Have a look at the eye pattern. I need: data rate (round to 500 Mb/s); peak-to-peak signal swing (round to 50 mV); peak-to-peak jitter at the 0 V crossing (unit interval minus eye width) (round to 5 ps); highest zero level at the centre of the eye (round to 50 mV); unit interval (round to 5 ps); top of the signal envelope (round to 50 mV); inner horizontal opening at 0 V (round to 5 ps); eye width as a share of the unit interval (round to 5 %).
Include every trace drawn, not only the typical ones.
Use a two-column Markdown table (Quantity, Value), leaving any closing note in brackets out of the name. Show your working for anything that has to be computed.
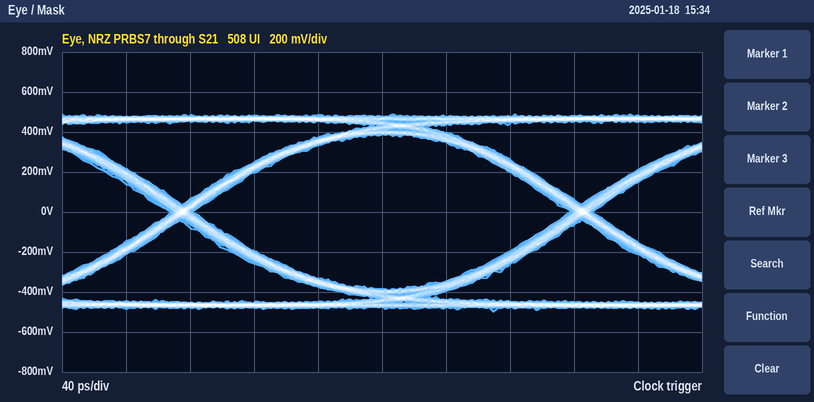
| Quantity | Value |
|---|---|
| data rate | 4.0 Gb/s |
| peak-to-peak signal swing | 1.00 V |
| peak-to-peak jitter at the 0 V crossing (unit interval minus eye width) | 15 ps |
| highest zero level at the centre of the eye | -400 mV |
| unit interval | 250 ps |
| top of the signal envelope | 500 mV |
| inner horizontal opening at 0 V | 235 ps |
| eye width as a share of the unit interval | 235 ps / 250 ps ≈ 94.0 %, so 95 % to the nearest 5 % |
